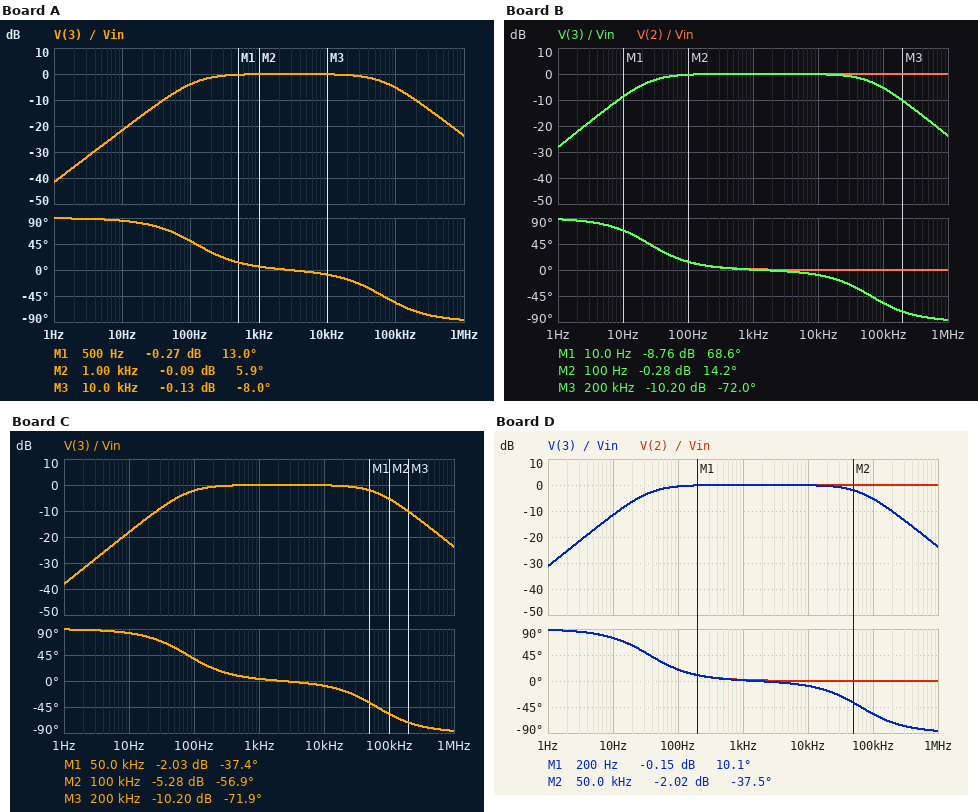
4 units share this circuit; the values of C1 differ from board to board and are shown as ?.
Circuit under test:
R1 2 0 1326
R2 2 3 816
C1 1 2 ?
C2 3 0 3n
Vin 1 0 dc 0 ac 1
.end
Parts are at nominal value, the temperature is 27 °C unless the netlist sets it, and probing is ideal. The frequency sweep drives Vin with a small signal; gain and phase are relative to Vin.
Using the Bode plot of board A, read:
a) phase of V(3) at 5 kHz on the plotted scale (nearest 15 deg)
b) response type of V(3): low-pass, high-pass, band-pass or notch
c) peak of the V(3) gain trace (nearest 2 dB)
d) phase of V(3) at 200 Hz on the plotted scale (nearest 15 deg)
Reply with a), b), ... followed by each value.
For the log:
a) 0 deg
b) band-pass
c) 0 dB
d) 30 deg
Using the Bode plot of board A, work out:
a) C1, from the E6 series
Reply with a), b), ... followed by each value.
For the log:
a) 1 µF
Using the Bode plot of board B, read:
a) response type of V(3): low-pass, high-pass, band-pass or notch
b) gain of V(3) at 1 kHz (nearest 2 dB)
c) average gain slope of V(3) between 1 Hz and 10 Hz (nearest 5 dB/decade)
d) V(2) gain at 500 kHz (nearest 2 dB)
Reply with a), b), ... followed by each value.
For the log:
a) band-pass
b) 0 dB
c) 20 dB/decade
d) 0 dB
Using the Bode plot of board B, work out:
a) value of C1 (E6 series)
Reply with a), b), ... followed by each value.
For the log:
a) 4.7 µF
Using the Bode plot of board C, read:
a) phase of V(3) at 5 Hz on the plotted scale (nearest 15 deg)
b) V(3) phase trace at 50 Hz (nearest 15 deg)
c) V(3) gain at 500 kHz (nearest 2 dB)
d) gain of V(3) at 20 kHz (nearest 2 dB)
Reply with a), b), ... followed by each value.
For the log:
a) 90 deg
b) 60 deg
c) -18 dB
d) 0 dB
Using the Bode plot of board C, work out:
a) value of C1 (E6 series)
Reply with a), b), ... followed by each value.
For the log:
a) 1.5 µF
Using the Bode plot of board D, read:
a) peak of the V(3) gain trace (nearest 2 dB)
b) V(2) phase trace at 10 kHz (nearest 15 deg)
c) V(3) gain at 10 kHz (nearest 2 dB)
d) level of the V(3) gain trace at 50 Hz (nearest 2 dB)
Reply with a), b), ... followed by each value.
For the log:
a) 0 dB
b) 0 deg
c) 0 dB
d) -2 dB
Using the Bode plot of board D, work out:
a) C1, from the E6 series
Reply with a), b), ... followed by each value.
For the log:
a) 3.3 µF
